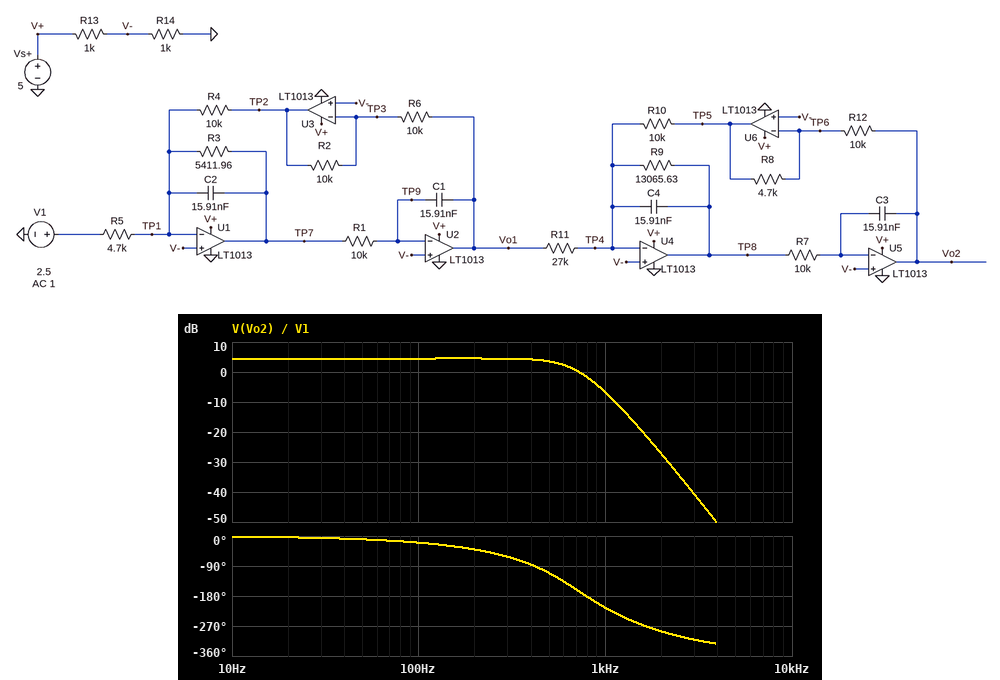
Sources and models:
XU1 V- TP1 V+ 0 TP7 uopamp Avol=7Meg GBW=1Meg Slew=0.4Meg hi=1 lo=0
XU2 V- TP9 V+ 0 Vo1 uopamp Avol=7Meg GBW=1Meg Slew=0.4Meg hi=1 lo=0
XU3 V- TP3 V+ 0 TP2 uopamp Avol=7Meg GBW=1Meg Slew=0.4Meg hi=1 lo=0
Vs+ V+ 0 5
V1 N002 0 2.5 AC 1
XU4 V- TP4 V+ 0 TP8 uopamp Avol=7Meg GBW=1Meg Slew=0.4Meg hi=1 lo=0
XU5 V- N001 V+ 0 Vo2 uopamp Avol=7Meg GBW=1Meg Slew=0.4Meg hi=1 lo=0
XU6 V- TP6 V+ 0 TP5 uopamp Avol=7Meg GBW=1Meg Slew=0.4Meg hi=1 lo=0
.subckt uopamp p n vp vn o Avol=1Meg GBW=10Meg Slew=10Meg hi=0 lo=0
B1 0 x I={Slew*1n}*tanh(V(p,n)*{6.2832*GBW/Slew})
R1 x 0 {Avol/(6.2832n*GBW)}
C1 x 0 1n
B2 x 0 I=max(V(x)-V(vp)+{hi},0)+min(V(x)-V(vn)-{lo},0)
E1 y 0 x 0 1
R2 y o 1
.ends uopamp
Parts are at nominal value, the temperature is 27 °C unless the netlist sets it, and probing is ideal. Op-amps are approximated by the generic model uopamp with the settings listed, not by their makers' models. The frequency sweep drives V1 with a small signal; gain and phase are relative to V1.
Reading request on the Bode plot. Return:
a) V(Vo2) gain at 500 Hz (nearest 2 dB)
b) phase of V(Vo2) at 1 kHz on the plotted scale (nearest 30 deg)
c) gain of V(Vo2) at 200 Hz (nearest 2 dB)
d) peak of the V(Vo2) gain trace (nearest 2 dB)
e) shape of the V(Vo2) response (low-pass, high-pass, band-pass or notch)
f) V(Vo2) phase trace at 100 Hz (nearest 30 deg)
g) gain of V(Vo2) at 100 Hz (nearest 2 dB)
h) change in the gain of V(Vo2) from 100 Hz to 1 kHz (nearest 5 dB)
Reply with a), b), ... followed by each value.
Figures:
a) 4 dB
b) -210 deg
c) 4 dB
d) 4 dB
e) low-pass
f) -30 deg
g) 4 dB
h) -10 dB
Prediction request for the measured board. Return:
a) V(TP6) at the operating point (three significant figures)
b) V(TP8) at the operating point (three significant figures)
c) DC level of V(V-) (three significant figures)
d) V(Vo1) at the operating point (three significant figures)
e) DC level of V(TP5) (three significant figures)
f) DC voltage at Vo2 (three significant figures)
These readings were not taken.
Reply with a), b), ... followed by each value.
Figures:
a) 2.50 V
b) 2.50 V
c) 2.50 V
d) 2.50 V
e) 2.50 V
f) 2.50 V
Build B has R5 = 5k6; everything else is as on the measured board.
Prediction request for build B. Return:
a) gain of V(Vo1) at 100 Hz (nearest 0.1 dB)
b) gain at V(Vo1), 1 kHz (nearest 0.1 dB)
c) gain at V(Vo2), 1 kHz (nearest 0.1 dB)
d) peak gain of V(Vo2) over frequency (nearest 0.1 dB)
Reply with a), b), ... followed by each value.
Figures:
a) 5.0 dB
b) -0.3 dB
c) -8.3 dB
d) 3.0 dB
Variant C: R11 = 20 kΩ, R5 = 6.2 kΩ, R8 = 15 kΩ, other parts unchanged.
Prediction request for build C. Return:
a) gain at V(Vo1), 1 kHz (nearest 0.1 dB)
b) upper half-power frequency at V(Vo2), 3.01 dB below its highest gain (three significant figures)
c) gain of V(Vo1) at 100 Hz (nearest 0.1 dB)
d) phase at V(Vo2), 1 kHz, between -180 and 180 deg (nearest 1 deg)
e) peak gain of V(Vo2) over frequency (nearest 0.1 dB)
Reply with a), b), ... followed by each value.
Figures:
a) -1.2 dB
b) 1.22 kHz
c) 4.1 dB
d) -147 deg
e) -5.4 dB
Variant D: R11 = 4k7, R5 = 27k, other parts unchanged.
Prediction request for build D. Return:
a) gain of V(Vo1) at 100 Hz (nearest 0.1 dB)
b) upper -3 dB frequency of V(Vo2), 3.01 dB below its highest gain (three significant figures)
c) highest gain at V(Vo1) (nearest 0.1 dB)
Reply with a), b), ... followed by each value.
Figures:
a) -8.7 dB
b) 650 Hz
c) -8.6 dB
